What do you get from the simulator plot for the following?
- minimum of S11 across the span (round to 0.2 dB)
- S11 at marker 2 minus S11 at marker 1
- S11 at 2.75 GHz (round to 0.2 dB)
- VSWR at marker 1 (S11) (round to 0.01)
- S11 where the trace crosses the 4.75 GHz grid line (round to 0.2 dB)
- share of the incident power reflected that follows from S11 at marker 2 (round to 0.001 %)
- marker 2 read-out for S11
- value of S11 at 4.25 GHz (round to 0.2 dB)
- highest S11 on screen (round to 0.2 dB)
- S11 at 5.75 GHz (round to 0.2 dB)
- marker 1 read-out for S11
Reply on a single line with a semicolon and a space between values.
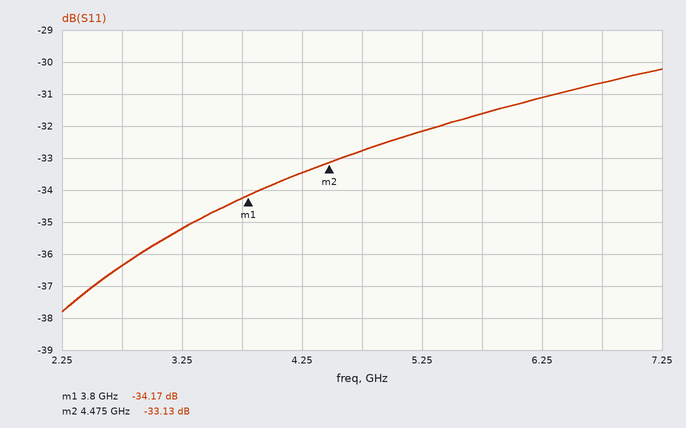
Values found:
-37.8 dB; 1.04 dB; -36.4 dB; 1.04; -32.8 dB; 0.049 %; -33.13 dB; -33.4 dB; -30.2 dB; -31.6 dB; -34.17 dB
